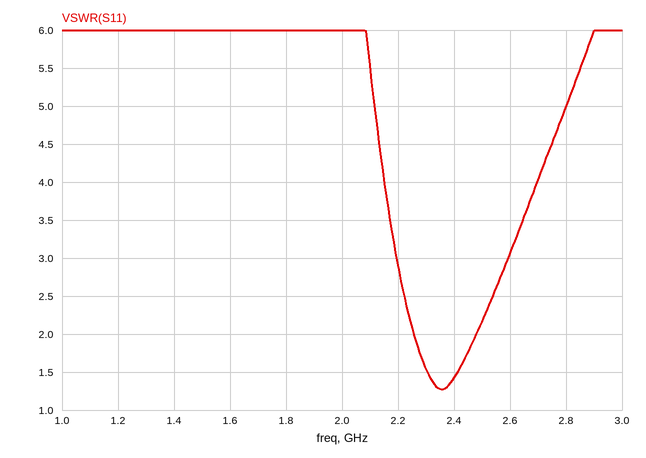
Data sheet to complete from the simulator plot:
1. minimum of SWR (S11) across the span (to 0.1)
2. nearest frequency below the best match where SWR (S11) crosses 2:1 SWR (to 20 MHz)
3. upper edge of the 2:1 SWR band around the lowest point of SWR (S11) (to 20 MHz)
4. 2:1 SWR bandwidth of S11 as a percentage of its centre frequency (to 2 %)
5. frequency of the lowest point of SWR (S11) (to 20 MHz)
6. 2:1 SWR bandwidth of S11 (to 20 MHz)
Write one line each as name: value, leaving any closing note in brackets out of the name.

minimum of SWR (S11) across the span: 1.3
nearest frequency below the best match where SWR (S11) crosses 2:1 SWR: 2.26 GHz
upper edge of the 2:1 SWR band around the lowest point of SWR (S11): 2.48 GHz
2:1 SWR bandwidth of S11 as a percentage of its centre frequency: 10 %
frequency of the lowest point of SWR (S11): 2.36 GHz
2:1 SWR bandwidth of S11: 220 MHz
